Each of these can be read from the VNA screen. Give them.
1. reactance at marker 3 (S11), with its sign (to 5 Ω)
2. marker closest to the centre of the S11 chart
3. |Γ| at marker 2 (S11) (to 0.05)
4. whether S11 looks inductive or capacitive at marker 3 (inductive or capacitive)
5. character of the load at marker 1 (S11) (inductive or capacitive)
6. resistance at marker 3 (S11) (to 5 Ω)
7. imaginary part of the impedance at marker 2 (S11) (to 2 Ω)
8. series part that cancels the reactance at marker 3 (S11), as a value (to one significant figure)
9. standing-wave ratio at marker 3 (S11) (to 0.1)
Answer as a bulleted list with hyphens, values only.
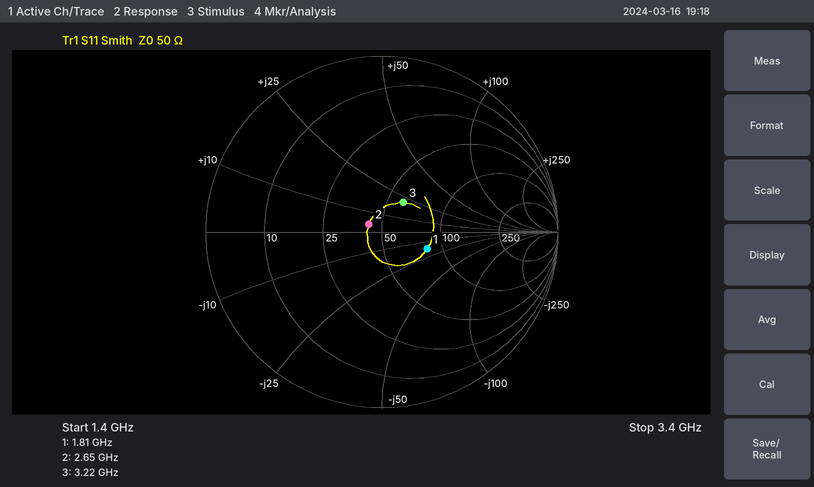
- +20 Ω
- marker 2
- 0.10
- inductive
- capacitive
- 60 Ω
- +4 Ω
- 2 pF
- 1.5
